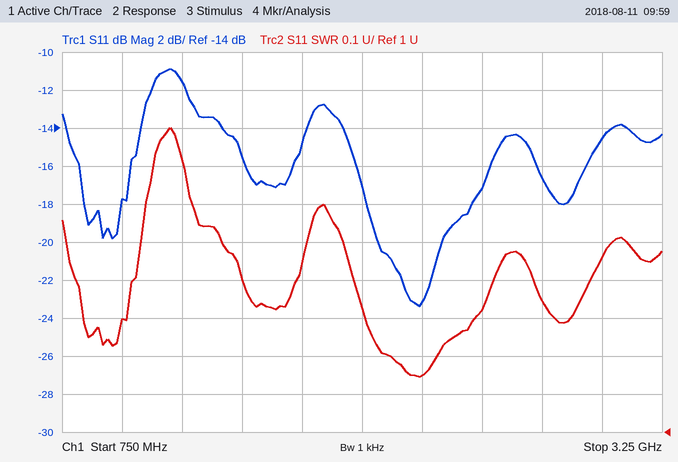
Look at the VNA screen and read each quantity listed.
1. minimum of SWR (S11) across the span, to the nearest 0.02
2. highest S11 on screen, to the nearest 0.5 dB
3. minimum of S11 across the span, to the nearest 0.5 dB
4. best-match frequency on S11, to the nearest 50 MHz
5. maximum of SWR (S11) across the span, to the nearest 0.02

1.14
-11.0 dB
-23.5 dB
2.25 GHz
1.80
